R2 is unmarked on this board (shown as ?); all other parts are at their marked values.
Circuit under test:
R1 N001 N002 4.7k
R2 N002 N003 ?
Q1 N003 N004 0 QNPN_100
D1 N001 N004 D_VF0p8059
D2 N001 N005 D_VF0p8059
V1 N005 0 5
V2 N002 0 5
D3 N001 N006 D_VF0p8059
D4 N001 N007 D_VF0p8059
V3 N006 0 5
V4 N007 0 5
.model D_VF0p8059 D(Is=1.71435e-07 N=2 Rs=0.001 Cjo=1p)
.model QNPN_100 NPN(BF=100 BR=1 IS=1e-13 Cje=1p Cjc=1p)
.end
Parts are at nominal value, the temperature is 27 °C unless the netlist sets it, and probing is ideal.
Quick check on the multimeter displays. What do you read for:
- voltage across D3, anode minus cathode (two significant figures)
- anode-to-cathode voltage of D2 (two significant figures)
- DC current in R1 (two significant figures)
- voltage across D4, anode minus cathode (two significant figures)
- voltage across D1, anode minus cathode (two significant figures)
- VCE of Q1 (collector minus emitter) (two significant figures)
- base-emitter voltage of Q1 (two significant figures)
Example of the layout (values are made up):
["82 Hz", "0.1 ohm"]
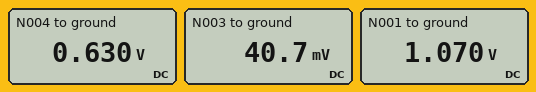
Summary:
["-3.9 V", "-3.9 V", "840 µA", "-3.9 V", "440 mV", "41 mV", "630 mV"]
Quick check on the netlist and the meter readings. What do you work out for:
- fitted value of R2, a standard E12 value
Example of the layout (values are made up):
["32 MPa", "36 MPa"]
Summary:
["2.2 kΩ"]
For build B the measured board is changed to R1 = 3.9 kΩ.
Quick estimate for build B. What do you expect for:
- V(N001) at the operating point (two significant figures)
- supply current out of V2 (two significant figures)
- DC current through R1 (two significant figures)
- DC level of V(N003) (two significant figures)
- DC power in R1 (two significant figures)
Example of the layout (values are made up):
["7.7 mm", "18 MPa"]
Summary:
["1.1 V", "3.3 mA", "1.0 mA", "38 mV", "3.9 mW"]
